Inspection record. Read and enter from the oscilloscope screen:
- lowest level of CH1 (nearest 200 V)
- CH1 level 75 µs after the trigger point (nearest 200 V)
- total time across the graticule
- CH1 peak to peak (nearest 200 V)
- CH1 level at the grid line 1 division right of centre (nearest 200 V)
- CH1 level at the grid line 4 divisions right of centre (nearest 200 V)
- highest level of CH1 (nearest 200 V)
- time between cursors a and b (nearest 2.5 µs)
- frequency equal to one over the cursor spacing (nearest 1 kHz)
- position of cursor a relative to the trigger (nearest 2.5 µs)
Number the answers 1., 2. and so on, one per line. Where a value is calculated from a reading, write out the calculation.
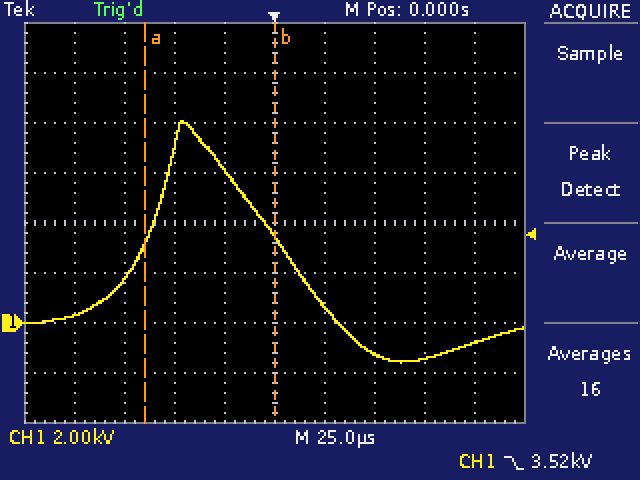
1. -1.6 kV
2. -1.4 kV
3. 250 µs
4. 8.0 kV − (-1.6 kV) = 9.6 kV
5. 600 V
6. -800 V
7. 8.0 kV
8. 65.0 µs
9. 1 / 65.0 µs ≈ 15 kHz
10. -65.0 µs
